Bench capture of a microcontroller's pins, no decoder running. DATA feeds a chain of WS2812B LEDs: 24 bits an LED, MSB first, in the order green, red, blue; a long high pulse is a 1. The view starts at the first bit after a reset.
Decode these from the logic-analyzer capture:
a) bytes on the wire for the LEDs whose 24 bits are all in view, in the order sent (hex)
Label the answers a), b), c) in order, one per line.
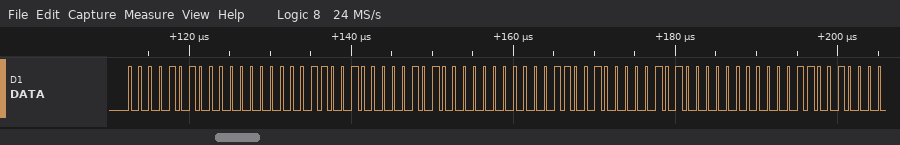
a) 0A 00 32 0A 00 32 0A 00 32
